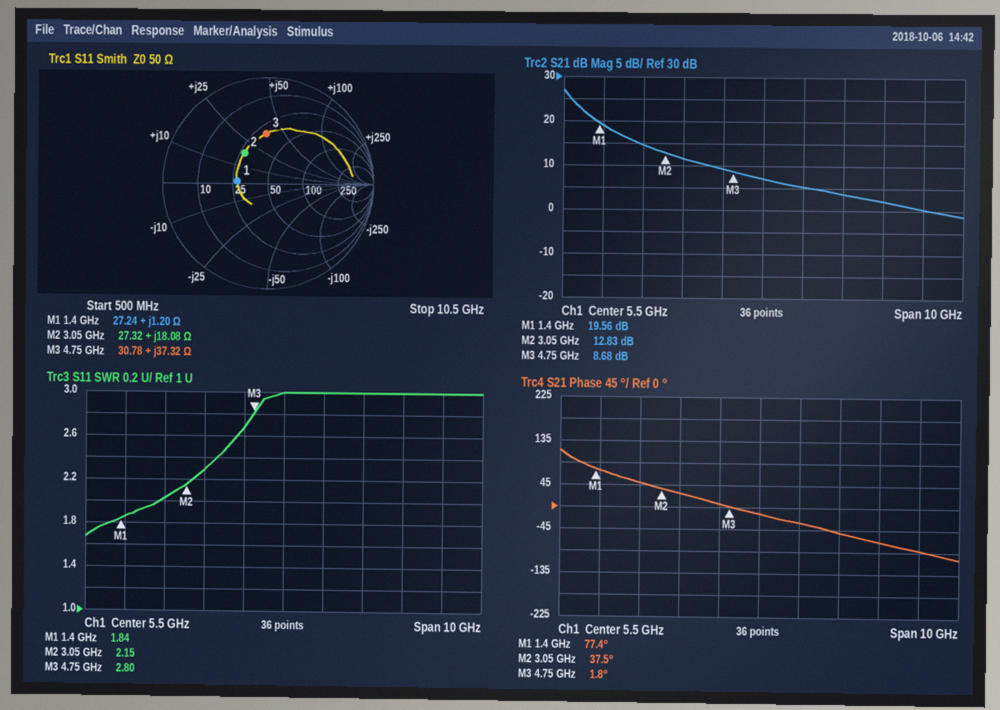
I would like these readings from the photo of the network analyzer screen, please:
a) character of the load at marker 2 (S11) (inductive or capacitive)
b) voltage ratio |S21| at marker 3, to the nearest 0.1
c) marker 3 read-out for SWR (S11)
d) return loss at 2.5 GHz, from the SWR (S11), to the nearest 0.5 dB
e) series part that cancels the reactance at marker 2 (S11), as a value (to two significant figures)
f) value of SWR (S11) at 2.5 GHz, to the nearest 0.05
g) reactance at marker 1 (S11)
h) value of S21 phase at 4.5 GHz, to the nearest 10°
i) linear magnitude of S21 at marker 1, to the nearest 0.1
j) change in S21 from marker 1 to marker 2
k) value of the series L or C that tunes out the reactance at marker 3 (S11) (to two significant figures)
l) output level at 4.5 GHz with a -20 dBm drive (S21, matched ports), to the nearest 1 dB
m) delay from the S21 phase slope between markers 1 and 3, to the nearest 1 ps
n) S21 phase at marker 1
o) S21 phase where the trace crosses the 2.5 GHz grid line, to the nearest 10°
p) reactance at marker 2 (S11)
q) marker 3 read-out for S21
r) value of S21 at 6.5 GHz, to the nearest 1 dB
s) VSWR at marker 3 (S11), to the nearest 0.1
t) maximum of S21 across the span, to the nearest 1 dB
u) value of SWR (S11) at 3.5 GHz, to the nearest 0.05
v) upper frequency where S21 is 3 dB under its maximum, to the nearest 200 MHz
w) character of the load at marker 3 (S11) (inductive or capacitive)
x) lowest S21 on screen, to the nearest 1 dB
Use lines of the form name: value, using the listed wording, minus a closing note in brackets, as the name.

character of the load at marker 2 (S11): inductive
voltage ratio |S21| at marker 3, to the nearest 0.1: 2.7
marker 3 read-out for SWR: 2.80
return loss at 2.5 GHz, from the SWR (S11), to the nearest 0.5 dB: 9.5 dB
series part that cancels the reactance at marker 2 (S11), as a value: 2.9 pF
value of SWR (S11) at 2.5 GHz, to the nearest 0.05: 2.05
reactance at marker 1: +1.20 Ω
value of S21 phase at 4.5 GHz, to the nearest 10°: 10°
linear magnitude of S21 at marker 1, to the nearest 0.1: 9.5
change in S21 from marker 1 to marker 2: -6.73 dB
value of the series L or C that tunes out the reactance at marker 3 (S11): 900 fF
output level at 4.5 GHz with a -20 dBm drive (S21, matched ports), to the nearest 1 dB: -11 dBm
delay from the S21 phase slope between markers 1 and 3, to the nearest 1 ps: 63 ps
S21 phase at marker 1: 77.4°
S21 phase where the trace crosses the 2.5 GHz grid line, to the nearest 10°: 50°
reactance at marker 2: +18.08 Ω
marker 3 read-out for S21: 8.68 dB
value of S21 at 6.5 GHz, to the nearest 1 dB: 5 dB
VSWR at marker 3 (S11), to the nearest 0.1: 2.8
maximum of S21 across the span, to the nearest 1 dB: 27 dB
value of SWR (S11) at 3.5 GHz, to the nearest 0.05: 2.30
upper frequency where S21 is 3 dB under its maximum, to the nearest 200 MHz: 800 MHz
character of the load at marker 3 (S11): inductive
lowest S21 on screen, to the nearest 1 dB: -1 dB
